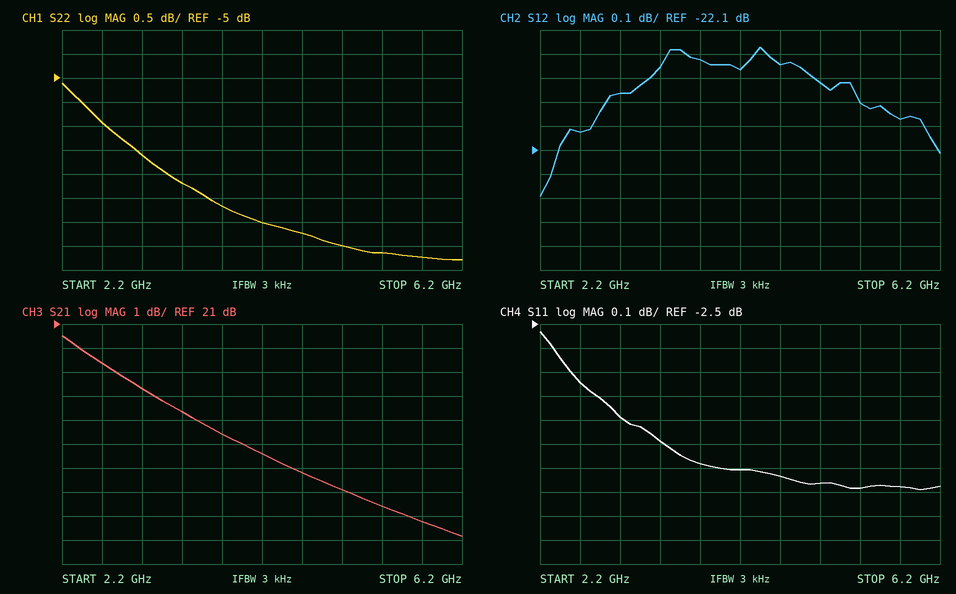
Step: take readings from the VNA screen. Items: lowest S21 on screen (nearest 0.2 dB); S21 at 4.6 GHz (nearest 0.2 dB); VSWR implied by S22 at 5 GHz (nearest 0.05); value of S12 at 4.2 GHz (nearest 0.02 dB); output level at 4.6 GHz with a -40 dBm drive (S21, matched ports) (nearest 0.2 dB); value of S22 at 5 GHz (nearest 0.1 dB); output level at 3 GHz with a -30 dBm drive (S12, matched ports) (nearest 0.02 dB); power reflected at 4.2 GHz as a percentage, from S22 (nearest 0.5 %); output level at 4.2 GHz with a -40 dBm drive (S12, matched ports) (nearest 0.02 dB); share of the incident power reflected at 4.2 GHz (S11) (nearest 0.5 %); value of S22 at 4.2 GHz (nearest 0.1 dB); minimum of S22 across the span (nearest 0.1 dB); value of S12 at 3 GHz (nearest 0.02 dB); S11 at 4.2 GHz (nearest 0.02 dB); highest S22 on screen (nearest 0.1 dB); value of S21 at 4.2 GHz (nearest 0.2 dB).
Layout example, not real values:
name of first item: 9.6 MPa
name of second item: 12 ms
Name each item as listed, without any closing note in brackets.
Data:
lowest S21 on screen: 12.2 dB
S21 at 4.6 GHz: 14.8 dB
VSWR implied by S22 at 5 GHz: 2.20
value of S12 at 4.2 GHz: -21.76 dB
output level at 4.6 GHz with a -40 dBm drive (S21, matched ports): -25.2 dBm
value of S22 at 5 GHz: -8.5 dB
output level at 3 GHz with a -30 dBm drive (S12, matched ports): -51.86 dBm
power reflected at 4.2 GHz as a percentage, from S22: 16.0 %
output level at 4.2 GHz with a -40 dBm drive (S12, matched ports): -61.76 dBm
share of the incident power reflected at 4.2 GHz (S11): 49.0 %
value of S22 at 4.2 GHz: -8.0 dB
minimum of S22 across the span: -8.8 dB
value of S12 at 3 GHz: -21.86 dB
S11 at 4.2 GHz: -3.10 dB
highest S22 on screen: -5.1 dB
value of S21 at 4.2 GHz: 15.6 dB
